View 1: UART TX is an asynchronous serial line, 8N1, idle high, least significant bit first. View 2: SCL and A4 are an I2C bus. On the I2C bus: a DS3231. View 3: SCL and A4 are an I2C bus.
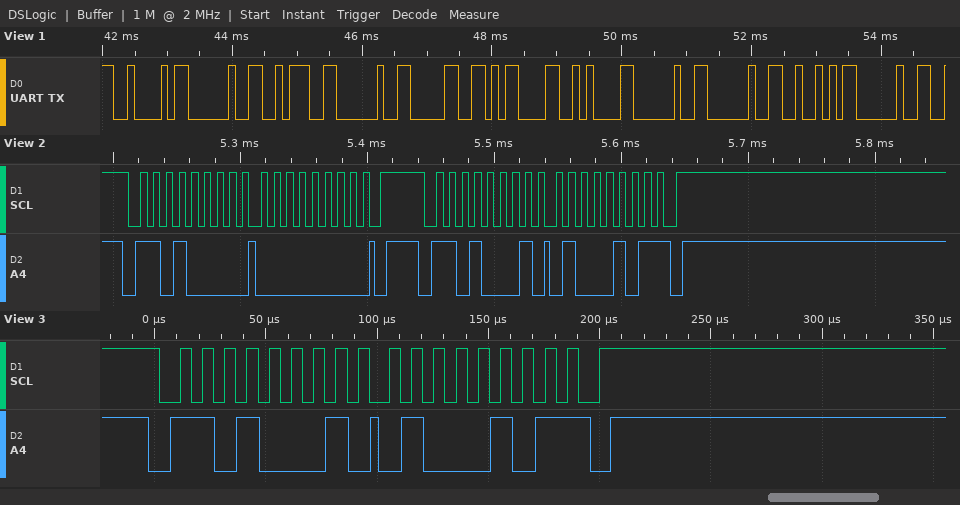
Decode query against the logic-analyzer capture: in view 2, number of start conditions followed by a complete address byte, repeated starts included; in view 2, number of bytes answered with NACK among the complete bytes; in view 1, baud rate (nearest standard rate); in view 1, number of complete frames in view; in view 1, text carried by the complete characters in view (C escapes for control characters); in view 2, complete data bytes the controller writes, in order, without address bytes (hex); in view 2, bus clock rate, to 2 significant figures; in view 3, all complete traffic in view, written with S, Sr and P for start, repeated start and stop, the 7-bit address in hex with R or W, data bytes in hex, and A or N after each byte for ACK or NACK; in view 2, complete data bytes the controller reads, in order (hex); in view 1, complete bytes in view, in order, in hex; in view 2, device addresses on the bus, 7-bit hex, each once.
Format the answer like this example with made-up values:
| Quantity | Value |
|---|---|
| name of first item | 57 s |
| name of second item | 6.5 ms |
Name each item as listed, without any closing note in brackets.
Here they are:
| Quantity | Value |
|---|---|
| in view 2, number of start conditions followed by a complete address byte, repeated starts included | 2 |
| in view 2, number of bytes answered with NACK among the complete bytes | 1 |
| in view 1, baud rate | 9600 baud |
| in view 1, number of complete frames in view | 11 |
| in view 1, text carried by the complete characters in view | "B : 0\r\n  R " |
| in view 2, complete data bytes the controller writes, in order, without address bytes | 00 |
| in view 2, bus clock rate, to 2 significant figures | 100 kHz |
| in view 3, all complete traffic in view, written with S, Sr and P for start, repeated start and stop, the 7-bit address in hex with R or W, data bytes in hex, and A or N after each byte for ACK or NACK | S 68R A 45 N P |
| in view 2, complete data bytes the controller reads, in order | 45 |
| in view 1, complete bytes in view, in order, in hex | 42 20 3A 20 30 0D 0A 20 20 52 20 |
| in view 2, device addresses on the bus, 7-bit hex, each once | 0x68 |
